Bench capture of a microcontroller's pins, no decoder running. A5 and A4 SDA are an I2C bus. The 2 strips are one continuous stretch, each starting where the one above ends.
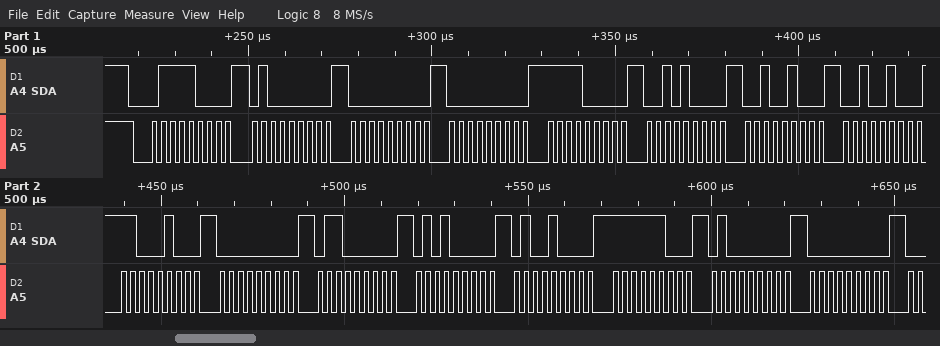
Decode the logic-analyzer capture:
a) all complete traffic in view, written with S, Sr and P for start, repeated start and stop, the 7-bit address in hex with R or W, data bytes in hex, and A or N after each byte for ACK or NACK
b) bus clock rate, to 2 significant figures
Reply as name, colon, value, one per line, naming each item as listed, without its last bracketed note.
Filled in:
all complete traffic in view, written with S, Sr and P for start, repeated start and stop, the 7-bit address in hex with R or W, data bytes in hex, and A or N after each byte for ACK or NACK: S 3CW A 40 A 00 A 00 A F0 A 28 A 24 A 24 A C4 A 00 A 60 A 50 A 48 A FC A 40 A 00 A
bus clock rate, to 2 significant figures: 400 kHz
